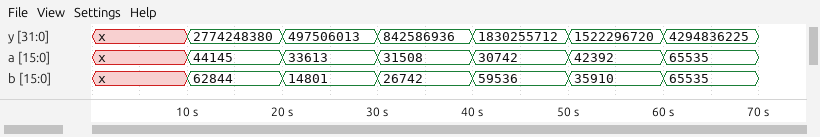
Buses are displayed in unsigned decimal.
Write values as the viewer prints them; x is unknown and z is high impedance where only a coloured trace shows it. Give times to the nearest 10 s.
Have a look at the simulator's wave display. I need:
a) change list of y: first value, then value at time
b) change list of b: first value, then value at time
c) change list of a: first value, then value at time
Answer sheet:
x, 2774248380 at 10 s, 497506013 at 20 s, 842586936 at 30 s, 1830255712 at 40 s, 1522296720 at 50 s, 4294836225 at 60 s
x, 62844 at 10 s, 14801 at 20 s, 26742 at 30 s, 59536 at 40 s, 35910 at 50 s, 65535 at 60 s
x, 44145 at 10 s, 33613 at 20 s, 31508 at 30 s, 30742 at 40 s, 42392 at 50 s, 65535 at 60 s
